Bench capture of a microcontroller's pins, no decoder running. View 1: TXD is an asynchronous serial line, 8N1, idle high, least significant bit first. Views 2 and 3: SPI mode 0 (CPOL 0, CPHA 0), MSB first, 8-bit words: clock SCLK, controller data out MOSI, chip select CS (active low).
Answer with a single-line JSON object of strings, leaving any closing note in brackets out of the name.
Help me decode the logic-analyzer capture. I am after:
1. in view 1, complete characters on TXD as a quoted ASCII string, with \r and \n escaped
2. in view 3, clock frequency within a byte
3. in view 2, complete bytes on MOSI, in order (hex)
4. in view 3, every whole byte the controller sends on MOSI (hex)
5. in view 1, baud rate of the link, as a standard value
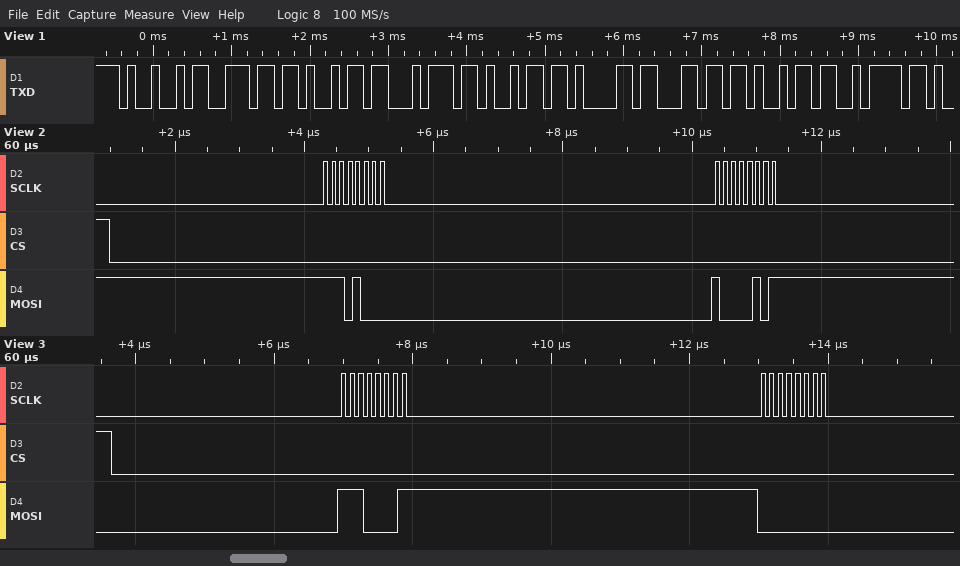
{"in view 1, complete characters on TXD as a quoted ASCII string, with \\r and \\n escaped": "\"Initializ\"", "in view 3, clock frequency within a byte": "8 MHz", "in view 2, complete bytes on MOSI, in order": "0xE8 0x85", "in view 3, every whole byte the controller sends on MOSI": "0xE1 0x00", "in view 1, baud rate of the link, as a standard value": "9600 baud"}
